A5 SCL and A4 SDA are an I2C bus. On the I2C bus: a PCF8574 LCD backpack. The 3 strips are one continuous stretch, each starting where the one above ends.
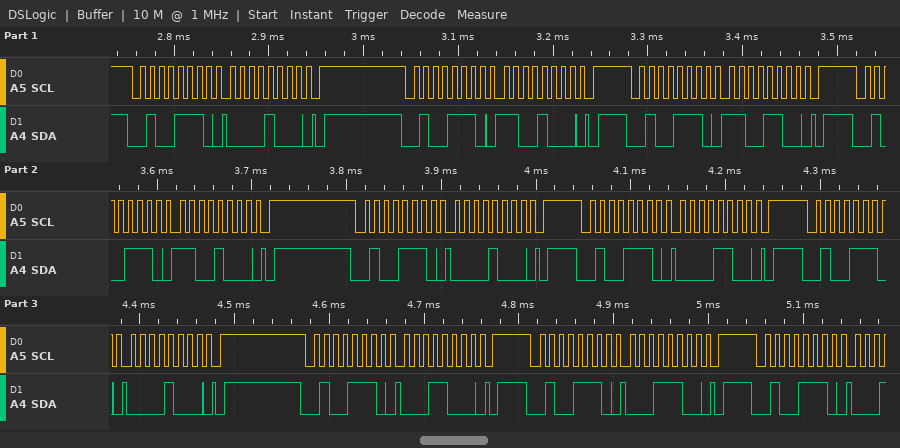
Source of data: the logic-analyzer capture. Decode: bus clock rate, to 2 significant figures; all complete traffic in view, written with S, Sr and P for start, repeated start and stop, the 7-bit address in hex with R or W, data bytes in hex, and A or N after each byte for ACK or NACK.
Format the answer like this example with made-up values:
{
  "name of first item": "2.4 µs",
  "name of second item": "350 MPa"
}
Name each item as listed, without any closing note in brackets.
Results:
{
  "bus clock rate, to 2 significant figures": "100 kHz",
  "all complete traffic in view, written with S, Sr and P for start, repeated start and stop, the 7-bit address in hex with R or W, data bytes in hex, and A or N after each byte for ACK or NACK": "S 27W A 08 A P S 27W A C8 A P S 27W A CC A P S 27W A C8 A P S 27W A 08 A P S 27W A 0C A P S 27W A 08 A P S 27W A 18 A P S 27W A 1C A P S 27W A"
}
